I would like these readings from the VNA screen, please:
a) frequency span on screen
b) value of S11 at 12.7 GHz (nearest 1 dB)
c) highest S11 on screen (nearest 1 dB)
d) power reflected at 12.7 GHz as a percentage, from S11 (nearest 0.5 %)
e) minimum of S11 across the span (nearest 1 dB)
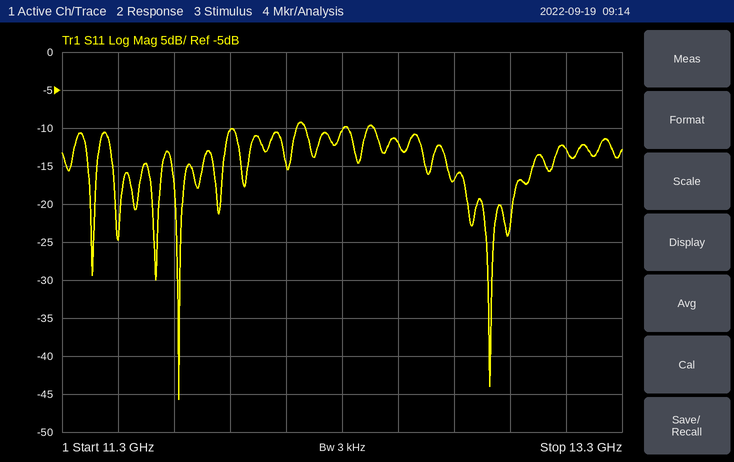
2 GHz
-17 dB
-9 dB
2.0 %
-46 dB
